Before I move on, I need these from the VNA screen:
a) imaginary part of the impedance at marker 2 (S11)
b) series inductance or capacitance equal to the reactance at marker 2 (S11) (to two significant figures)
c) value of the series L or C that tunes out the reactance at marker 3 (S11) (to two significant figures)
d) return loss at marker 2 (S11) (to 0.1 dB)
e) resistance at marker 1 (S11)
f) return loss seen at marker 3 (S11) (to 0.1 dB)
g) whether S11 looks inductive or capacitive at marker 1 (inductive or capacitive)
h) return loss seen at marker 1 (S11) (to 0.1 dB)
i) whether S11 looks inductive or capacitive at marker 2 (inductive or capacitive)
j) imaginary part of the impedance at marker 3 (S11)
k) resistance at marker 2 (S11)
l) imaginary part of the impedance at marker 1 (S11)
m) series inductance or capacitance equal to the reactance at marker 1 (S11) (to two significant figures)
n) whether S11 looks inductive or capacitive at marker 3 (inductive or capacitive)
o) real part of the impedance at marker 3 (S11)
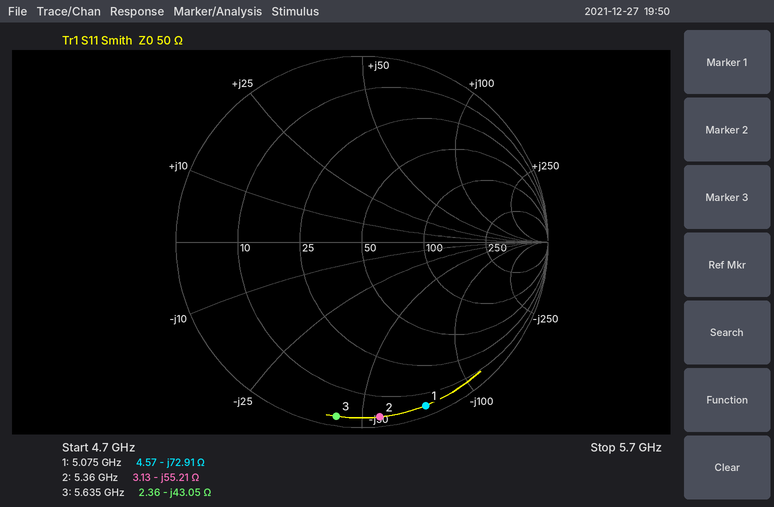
-55.21 Ω
540 fF
1.2 nH
0.5 dB
4.57 Ω
0.5 dB
capacitive
0.5 dB
capacitive
-43.05 Ω
3.13 Ω
-72.91 Ω
430 fF
capacitive
2.36 Ω
